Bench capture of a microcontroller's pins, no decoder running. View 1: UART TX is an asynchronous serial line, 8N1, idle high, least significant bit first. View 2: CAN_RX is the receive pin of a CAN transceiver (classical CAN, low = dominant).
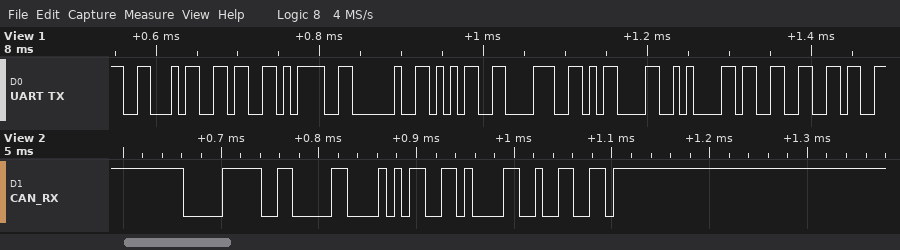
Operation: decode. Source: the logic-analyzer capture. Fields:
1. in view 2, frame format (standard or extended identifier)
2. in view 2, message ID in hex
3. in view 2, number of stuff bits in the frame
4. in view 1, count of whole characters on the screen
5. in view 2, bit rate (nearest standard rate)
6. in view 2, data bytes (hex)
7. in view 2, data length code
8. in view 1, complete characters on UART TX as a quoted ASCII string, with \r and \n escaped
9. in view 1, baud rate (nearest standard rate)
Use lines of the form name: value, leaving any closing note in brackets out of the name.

in view 2, frame format: standard
in view 2, message ID in hex: 0x07B
in view 2, number of stuff bits in the frame: 3
in view 1, count of whole characters on the screen: 10
in view 2, bit rate: 125 kbit/s
in view 2, data bytes: 15 9A
in view 2, data length code: 2
in view 1, complete characters on UART TX as a quoted ASCII string, with \r and \n escaped: "F6= 58\r\n36"
in view 1, baud rate: 115200 baud
